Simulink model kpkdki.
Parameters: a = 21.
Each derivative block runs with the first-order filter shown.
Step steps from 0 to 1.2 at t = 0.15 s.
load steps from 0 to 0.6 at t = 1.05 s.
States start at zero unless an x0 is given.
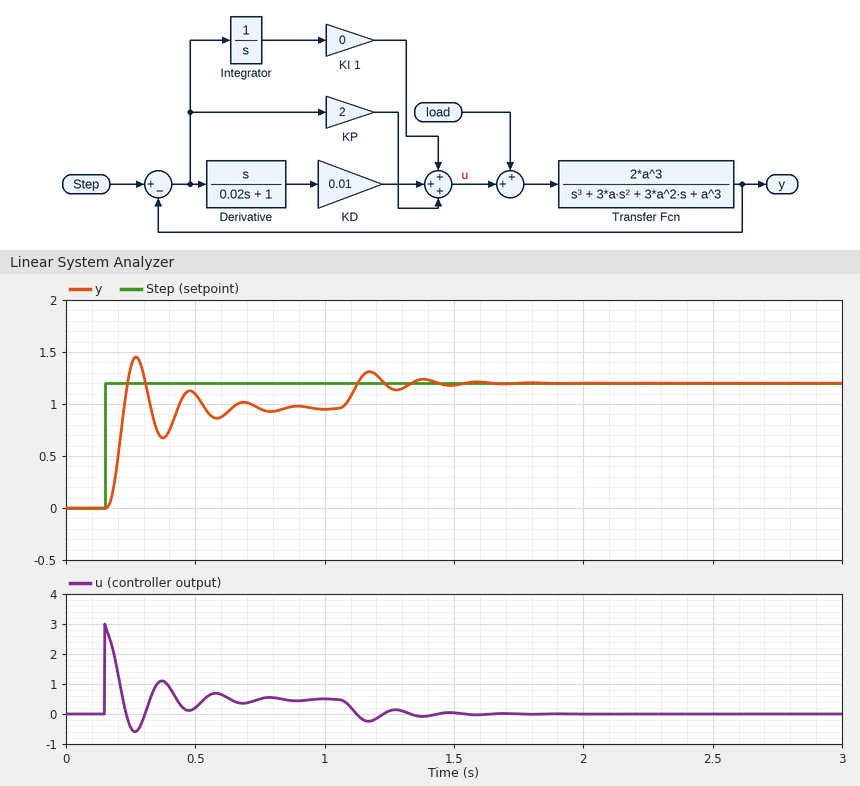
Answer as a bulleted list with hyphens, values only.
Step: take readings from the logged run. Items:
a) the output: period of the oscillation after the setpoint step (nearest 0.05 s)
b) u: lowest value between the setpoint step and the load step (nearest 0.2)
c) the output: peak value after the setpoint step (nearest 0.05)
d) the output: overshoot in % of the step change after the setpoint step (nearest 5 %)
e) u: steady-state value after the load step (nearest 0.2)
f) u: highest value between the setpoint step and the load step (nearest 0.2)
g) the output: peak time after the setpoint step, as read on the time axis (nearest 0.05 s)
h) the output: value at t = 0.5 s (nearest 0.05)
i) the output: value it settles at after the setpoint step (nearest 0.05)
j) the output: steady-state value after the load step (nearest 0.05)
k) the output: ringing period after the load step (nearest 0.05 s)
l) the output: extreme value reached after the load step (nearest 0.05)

- 0.20 s
- -0.6
- 1.45
- 50 %
- 0.0
- 3.0
- 0.25 s
- 1.10
- 0.95
- 1.20
- 0.20 s
- 1.30
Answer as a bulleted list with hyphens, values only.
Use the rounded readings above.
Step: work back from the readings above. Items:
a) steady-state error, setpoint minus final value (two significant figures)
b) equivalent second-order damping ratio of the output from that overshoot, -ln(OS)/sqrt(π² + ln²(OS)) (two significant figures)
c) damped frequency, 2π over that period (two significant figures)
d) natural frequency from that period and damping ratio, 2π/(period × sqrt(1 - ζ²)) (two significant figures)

- 0.25
- 0.22
- 31 rad/s
- 32 rad/s
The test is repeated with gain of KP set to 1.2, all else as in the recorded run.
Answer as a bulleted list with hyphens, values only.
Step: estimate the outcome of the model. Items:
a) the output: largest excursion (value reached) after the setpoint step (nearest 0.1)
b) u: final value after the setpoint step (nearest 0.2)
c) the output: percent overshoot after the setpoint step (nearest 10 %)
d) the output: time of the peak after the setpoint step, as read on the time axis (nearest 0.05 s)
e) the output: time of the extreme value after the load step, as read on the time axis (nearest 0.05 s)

- 1.1
- 0.4
- 30 %
- 0.30 s
- 1.20 s
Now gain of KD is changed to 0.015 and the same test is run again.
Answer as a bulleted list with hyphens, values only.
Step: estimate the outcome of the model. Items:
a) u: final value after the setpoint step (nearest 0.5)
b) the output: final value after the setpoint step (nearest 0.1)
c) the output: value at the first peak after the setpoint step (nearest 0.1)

- 0.5
- 1.0
- 1.4
